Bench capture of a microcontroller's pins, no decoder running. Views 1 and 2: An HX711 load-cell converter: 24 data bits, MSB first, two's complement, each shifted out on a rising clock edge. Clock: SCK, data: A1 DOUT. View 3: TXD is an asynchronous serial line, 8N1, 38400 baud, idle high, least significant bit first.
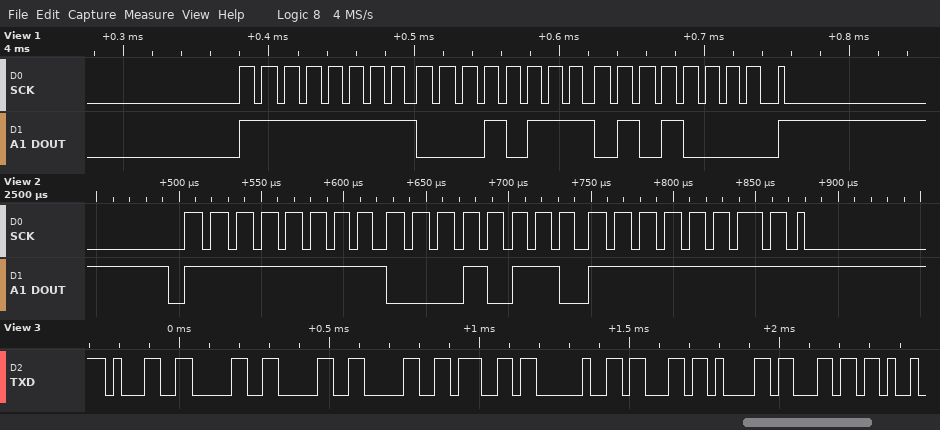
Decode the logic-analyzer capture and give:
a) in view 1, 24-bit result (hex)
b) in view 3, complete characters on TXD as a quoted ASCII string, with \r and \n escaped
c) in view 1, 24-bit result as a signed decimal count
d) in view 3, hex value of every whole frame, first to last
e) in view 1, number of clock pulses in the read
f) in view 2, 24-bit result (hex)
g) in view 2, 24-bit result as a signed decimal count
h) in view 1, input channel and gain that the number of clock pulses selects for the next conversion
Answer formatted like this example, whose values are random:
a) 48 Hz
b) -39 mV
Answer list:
a) 0xFF1750
b) "1000g cal"
c) -59568
d) 31 30 30 30 67 20 63 61 6C
e) 25
f) 0xFF16FF
g) -59649
h) channel A, gain 128
